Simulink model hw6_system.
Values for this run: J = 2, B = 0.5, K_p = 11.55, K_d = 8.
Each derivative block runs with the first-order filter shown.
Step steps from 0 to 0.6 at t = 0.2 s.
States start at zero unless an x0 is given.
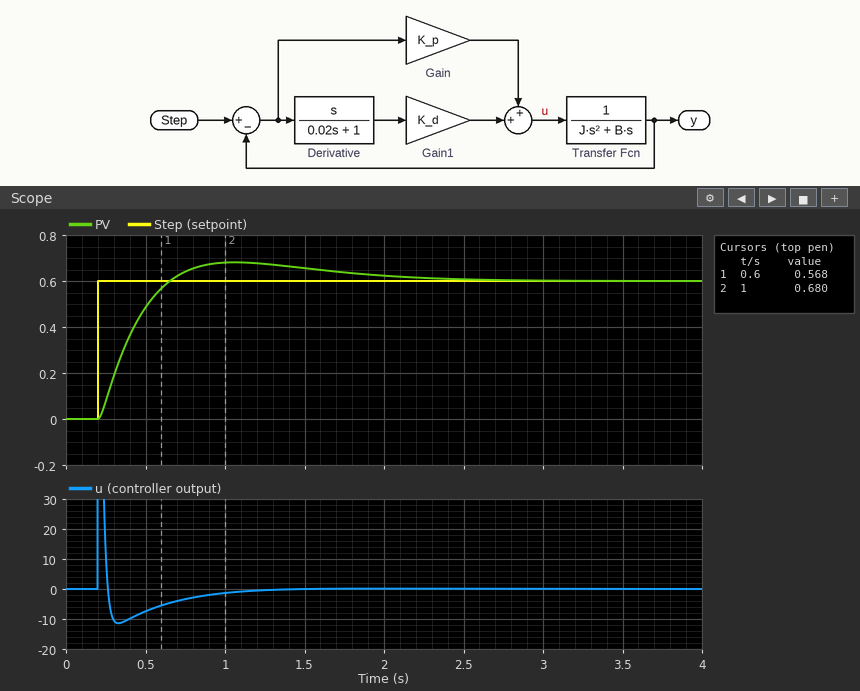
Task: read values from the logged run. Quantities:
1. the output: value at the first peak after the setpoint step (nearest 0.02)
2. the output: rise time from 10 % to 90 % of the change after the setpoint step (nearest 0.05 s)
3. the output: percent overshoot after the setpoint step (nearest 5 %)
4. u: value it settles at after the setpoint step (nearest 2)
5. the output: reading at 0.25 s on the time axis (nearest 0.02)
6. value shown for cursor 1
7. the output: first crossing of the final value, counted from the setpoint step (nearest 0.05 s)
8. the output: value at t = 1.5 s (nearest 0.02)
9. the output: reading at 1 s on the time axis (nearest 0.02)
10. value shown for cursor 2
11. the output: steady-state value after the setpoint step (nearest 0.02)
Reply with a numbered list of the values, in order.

1. 0.68
2. 0.30 s
3. 15 %
4. 0
5. 0.08
6. 0.568
7. 0.45 s
8. 0.66
9. 0.68
10. 0.680
11. 0.60
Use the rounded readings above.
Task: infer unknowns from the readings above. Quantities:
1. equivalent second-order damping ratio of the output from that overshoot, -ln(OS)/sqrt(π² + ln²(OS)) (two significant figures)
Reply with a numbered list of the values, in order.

1. 0.52
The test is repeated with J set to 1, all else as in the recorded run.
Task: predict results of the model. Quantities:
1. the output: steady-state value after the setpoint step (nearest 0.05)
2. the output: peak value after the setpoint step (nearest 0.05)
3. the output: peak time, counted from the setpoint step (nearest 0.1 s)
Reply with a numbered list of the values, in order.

1. 0.60
2. 0.65
3. 0.5 s
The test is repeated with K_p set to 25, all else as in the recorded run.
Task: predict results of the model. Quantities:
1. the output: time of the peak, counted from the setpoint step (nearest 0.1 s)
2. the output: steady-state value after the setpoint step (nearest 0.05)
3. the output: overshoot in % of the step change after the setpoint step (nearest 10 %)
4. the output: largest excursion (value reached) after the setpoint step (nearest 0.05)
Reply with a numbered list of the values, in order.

1. 0.6 s
2. 0.60
3. 20 %
4. 0.75
